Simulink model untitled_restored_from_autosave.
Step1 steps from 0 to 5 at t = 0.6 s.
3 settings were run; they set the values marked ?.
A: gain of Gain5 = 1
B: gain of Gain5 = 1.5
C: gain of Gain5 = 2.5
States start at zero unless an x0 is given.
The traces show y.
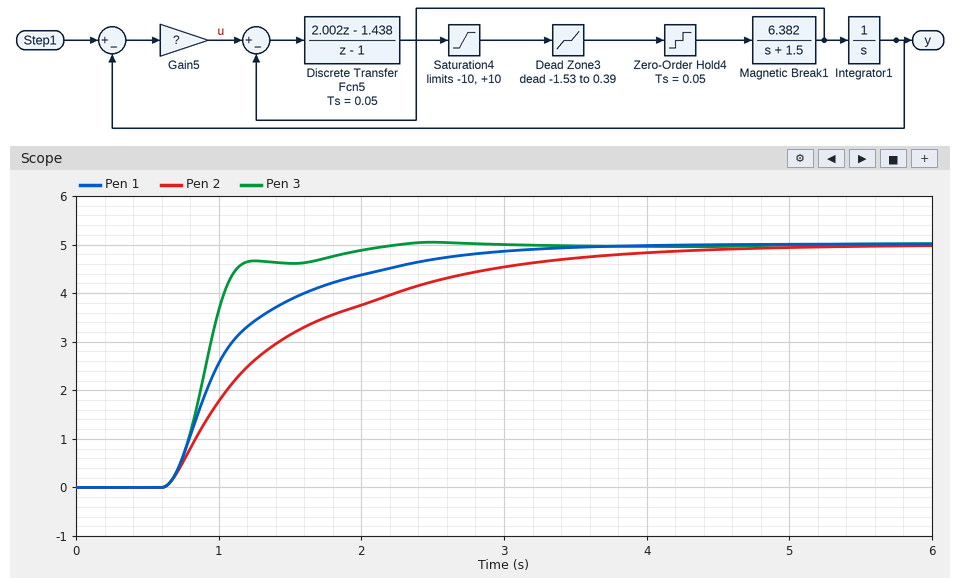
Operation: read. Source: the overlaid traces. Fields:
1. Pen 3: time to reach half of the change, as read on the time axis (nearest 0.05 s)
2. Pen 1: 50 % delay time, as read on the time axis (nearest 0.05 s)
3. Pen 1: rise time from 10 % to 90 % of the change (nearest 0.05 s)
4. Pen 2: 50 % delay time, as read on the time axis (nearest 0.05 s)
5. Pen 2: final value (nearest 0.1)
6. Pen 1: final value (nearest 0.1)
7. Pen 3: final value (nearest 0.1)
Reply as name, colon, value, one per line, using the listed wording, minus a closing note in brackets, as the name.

Pen 3: time to reach half of the change, as read on the time axis: 0.90 s
Pen 1: 50 % delay time, as read on the time axis: 1.00 s
Pen 1: rise time from 10 % to 90 % of the change: 1.45 s
Pen 2: 50 % delay time, as read on the time axis: 1.20 s
Pen 2: final value: 5.0
Pen 1: final value: 5.0
Pen 3: final value: 5.0
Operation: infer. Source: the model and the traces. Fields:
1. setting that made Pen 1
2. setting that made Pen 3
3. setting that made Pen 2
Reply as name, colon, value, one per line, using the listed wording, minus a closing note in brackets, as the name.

setting that made Pen 1: B
setting that made Pen 3: C
setting that made Pen 2: A
